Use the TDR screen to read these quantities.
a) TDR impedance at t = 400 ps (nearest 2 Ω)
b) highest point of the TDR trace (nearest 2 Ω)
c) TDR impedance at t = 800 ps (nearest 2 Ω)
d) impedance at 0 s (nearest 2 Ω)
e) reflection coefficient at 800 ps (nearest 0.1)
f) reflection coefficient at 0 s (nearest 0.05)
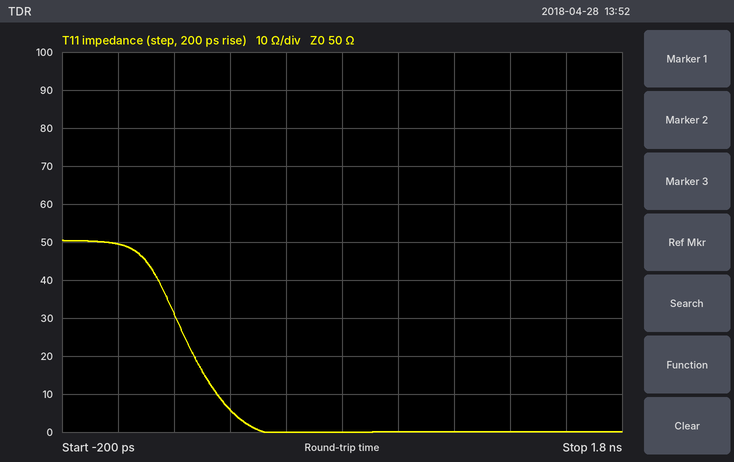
6 Ω
50 Ω
0 Ω
50 Ω
-1.0
0.00
